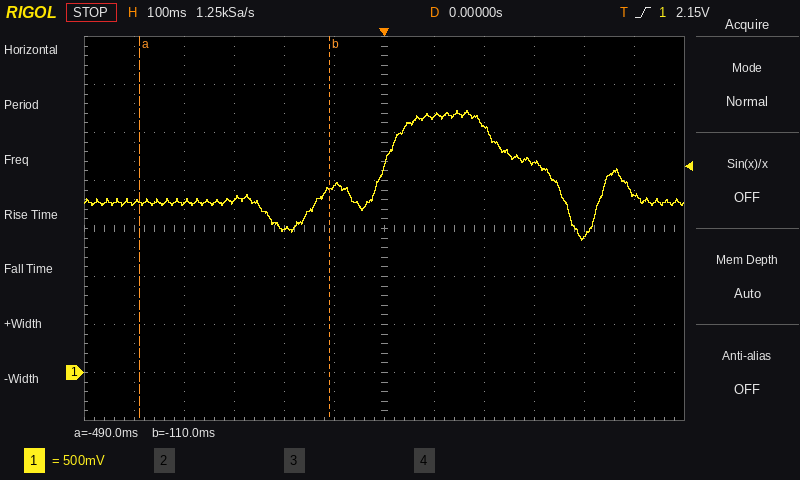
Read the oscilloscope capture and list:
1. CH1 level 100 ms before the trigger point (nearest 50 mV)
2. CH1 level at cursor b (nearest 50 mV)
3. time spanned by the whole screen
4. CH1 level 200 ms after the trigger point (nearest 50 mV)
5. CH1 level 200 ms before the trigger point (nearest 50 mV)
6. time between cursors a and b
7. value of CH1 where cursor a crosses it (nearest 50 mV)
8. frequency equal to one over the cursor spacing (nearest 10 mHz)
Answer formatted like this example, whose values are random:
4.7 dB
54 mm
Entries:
1.95 V
1.90 V
1.2 s
2.55 V
1.50 V
380 ms
1.75 V
2.63 Hz
